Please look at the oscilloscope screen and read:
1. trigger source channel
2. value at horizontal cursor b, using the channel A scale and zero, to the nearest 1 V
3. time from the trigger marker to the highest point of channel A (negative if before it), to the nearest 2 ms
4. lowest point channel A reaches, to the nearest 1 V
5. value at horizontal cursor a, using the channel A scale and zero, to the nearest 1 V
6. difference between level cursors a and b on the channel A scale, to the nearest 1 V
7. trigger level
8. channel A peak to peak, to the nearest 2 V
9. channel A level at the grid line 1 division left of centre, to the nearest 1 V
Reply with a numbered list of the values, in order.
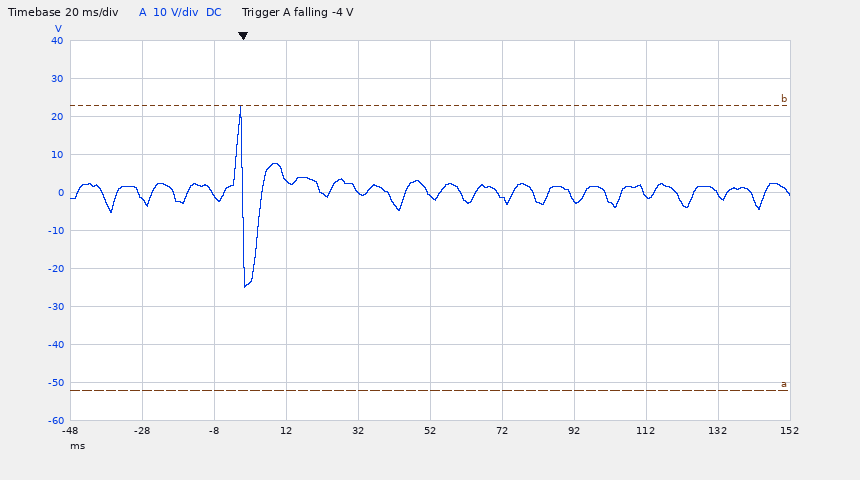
1. channel A
2. 23 V
3. 0 ms
4. -25 V
5. -52 V
6. 75 V
7. -4 V
8. 48 V
9. 0 V
